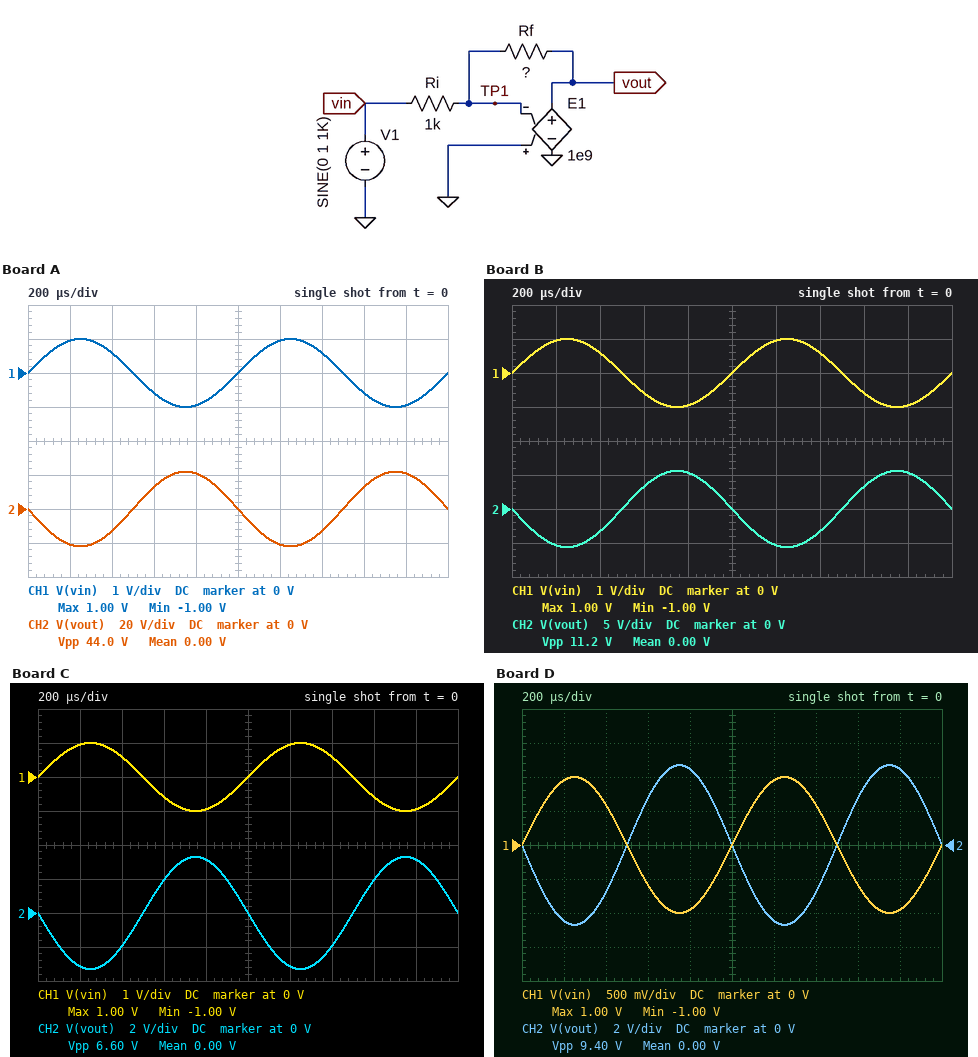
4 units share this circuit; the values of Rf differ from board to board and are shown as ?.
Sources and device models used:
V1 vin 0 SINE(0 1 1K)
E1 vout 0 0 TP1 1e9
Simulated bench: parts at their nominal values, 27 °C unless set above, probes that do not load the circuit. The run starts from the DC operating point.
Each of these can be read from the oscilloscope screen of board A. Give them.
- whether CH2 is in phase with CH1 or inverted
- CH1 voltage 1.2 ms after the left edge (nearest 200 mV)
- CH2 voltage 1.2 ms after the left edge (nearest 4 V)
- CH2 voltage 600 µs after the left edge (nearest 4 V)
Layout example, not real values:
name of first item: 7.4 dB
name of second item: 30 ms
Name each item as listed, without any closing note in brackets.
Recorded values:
whether CH2 is in phase with CH1 or inverted: inverted
CH1 voltage 1.2 ms after the left edge: 1.0 V
CH2 voltage 1.2 ms after the left edge: -20 V
CH2 voltage 600 µs after the left edge: 12 V
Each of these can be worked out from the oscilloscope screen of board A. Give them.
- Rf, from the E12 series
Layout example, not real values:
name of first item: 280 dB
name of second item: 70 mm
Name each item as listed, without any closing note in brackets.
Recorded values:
Rf, from the E12 series: 22 kΩ
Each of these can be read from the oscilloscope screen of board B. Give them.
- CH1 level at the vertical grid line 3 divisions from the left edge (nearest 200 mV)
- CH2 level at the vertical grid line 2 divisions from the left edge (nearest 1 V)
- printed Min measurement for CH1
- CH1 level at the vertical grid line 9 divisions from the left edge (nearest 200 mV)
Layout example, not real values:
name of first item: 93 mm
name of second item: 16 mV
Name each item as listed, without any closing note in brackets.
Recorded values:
CH1 level at the vertical grid line 3 divisions from the left edge: -600 mV
CH2 level at the vertical grid line 2 divisions from the left edge: -3 V
printed Min measurement for CH1: -1.00 V
CH1 level at the vertical grid line 9 divisions from the left edge: -1.0 V
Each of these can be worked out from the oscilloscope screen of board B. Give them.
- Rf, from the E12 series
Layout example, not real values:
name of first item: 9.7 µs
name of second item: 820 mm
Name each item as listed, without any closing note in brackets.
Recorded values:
Rf, from the E12 series: 5.6 kΩ
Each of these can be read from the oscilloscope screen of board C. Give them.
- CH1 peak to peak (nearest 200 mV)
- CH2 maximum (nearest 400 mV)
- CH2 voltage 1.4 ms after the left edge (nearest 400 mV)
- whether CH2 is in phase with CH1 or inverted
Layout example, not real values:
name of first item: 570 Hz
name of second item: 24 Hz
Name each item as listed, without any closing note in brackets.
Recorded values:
CH1 peak to peak: 2.0 V
CH2 maximum: 3.2 V
CH2 voltage 1.4 ms after the left edge: -2.0 V
whether CH2 is in phase with CH1 or inverted: inverted
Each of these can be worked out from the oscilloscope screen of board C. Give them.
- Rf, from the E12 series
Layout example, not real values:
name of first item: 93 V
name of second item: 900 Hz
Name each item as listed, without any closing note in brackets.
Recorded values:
Rf, from the E12 series: 3.3 kΩ
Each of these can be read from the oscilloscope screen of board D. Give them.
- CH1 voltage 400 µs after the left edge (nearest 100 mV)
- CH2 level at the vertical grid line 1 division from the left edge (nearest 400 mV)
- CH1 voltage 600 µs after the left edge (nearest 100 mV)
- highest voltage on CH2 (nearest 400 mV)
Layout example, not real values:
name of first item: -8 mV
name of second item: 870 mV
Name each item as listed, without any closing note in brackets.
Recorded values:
CH1 voltage 400 µs after the left edge: 600 mV
CH2 level at the vertical grid line 1 division from the left edge: -4.4 V
CH1 voltage 600 µs after the left edge: -600 mV
highest voltage on CH2: 4.8 V
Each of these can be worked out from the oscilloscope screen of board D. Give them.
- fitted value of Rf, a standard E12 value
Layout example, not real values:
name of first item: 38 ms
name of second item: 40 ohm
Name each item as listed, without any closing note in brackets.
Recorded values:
fitted value of Rf, a standard E12 value: 4.7 kΩ
